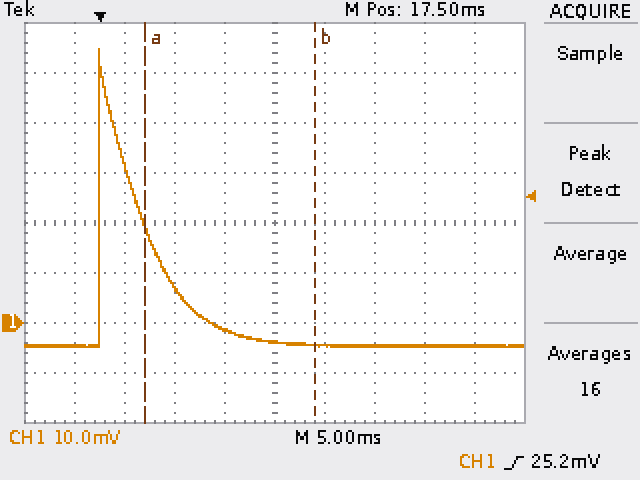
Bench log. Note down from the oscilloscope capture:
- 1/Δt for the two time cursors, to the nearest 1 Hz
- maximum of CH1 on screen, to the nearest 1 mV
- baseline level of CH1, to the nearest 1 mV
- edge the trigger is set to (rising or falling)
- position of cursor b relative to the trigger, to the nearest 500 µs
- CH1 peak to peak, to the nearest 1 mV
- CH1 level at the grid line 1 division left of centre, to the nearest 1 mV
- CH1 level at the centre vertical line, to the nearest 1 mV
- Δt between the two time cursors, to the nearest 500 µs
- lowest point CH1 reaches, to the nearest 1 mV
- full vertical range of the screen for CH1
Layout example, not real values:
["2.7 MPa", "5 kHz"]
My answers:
["59 Hz", "55 mV", "-5 mV", "rising", "+21.5 ms", "60 mV", "-1 mV", "-4 mV", "17.0 ms", "-5 mV", "80 mV"]
